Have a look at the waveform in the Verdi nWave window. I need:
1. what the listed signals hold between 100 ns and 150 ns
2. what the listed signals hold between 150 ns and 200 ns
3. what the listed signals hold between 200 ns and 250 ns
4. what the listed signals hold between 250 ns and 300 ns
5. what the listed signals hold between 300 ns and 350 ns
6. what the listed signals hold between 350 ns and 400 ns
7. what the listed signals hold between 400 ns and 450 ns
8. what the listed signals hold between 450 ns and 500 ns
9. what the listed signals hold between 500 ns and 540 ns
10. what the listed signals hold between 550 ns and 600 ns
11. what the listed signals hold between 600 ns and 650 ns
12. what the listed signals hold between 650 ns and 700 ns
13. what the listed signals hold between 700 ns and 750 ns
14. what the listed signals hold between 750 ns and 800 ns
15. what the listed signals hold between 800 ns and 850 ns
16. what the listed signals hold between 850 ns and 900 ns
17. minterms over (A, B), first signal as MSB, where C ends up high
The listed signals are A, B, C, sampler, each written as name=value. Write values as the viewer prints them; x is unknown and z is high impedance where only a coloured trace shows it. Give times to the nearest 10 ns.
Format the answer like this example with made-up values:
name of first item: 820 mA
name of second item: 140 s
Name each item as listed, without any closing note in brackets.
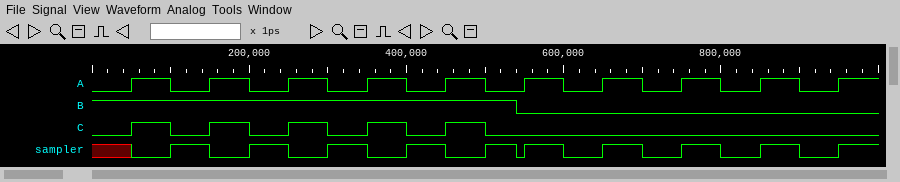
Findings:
what the listed signals hold between 100 ns and 150 ns: A=0, B=1, C=0, sampler=1
what the listed signals hold between 150 ns and 200 ns: A=1, B=1, C=1, sampler=0
what the listed signals hold between 200 ns and 250 ns: A=0, B=1, C=0, sampler=1
what the listed signals hold between 250 ns and 300 ns: A=1, B=1, C=1, sampler=0
what the listed signals hold between 300 ns and 350 ns: A=0, B=1, C=0, sampler=1
what the listed signals hold between 350 ns and 400 ns: A=1, B=1, C=1, sampler=0
what the listed signals hold between 400 ns and 450 ns: A=0, B=1, C=0, sampler=1
what the listed signals hold between 450 ns and 500 ns: A=1, B=1, C=1, sampler=0
what the listed signals hold between 500 ns and 540 ns: A=0, B=1, C=0, sampler=1
what the listed signals hold between 550 ns and 600 ns: A=1, B=0, C=0, sampler=1
what the listed signals hold between 600 ns and 650 ns: A=0, B=0, C=0, sampler=0
what the listed signals hold between 650 ns and 700 ns: A=1, B=0, C=0, sampler=1
what the listed signals hold between 700 ns and 750 ns: A=0, B=0, C=0, sampler=0
what the listed signals hold between 750 ns and 800 ns: A=1, B=0, C=0, sampler=1
what the listed signals hold between 800 ns and 850 ns: A=0, B=0, C=0, sampler=0
what the listed signals hold between 850 ns and 900 ns: A=1, B=0, C=0, sampler=1
minterms over (A, B), first signal as MSB, where C ends up high: 3
